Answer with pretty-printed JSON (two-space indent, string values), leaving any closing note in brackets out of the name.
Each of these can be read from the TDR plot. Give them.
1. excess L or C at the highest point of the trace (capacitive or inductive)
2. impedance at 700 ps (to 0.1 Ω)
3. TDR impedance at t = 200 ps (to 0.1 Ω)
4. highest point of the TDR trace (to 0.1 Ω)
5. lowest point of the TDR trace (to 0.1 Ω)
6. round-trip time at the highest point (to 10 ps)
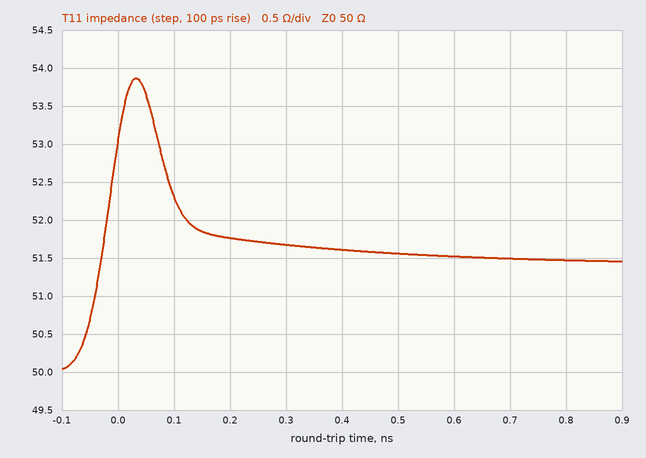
{
  "excess L or C at the highest point of the trace": "inductive",
  "impedance at 700 ps": "51.5 Ω",
  "TDR impedance at t = 200 ps": "51.8 Ω",
  "highest point of the TDR trace": "53.9 Ω",
  "lowest point of the TDR trace": "50.0 Ω",
  "round-trip time at the highest point": "30 ps"
}
